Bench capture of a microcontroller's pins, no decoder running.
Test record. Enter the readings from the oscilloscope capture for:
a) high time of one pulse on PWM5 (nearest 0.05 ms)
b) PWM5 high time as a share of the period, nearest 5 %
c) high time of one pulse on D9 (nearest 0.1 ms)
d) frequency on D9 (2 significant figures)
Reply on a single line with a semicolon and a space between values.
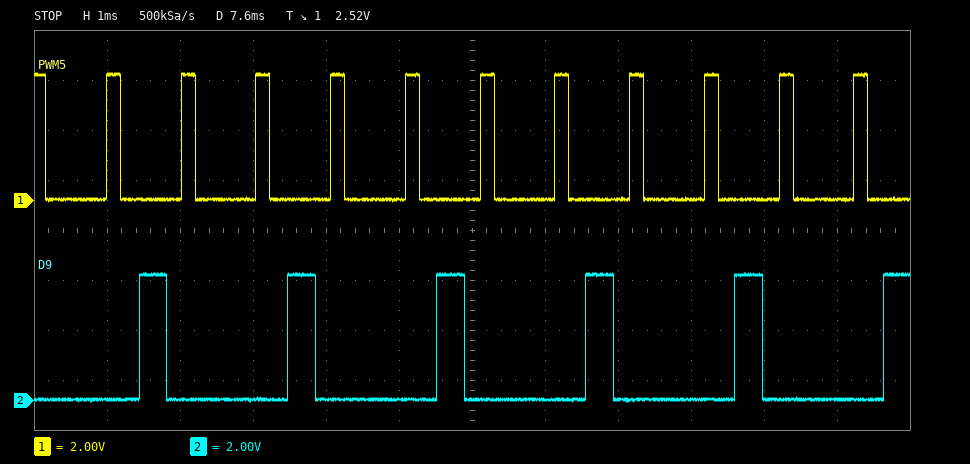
0.20 ms; 20 %; 0.4 ms; 490 Hz
